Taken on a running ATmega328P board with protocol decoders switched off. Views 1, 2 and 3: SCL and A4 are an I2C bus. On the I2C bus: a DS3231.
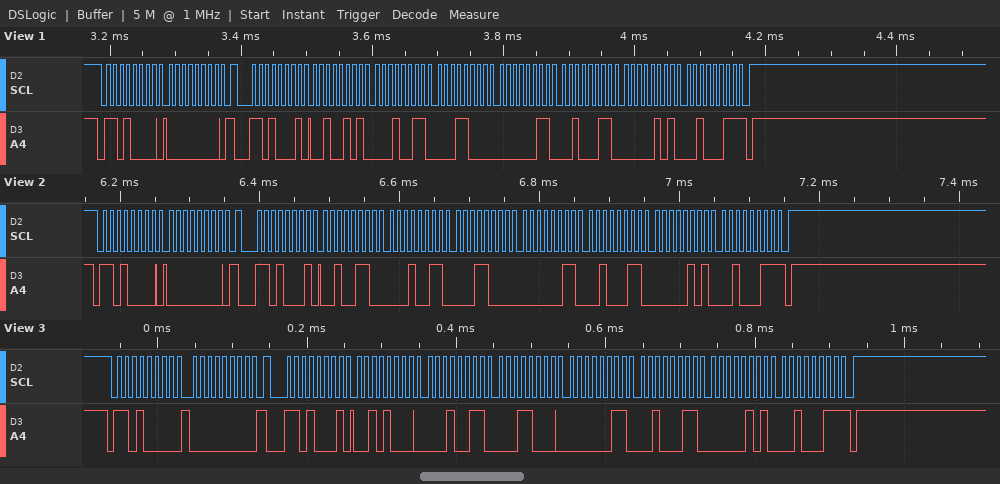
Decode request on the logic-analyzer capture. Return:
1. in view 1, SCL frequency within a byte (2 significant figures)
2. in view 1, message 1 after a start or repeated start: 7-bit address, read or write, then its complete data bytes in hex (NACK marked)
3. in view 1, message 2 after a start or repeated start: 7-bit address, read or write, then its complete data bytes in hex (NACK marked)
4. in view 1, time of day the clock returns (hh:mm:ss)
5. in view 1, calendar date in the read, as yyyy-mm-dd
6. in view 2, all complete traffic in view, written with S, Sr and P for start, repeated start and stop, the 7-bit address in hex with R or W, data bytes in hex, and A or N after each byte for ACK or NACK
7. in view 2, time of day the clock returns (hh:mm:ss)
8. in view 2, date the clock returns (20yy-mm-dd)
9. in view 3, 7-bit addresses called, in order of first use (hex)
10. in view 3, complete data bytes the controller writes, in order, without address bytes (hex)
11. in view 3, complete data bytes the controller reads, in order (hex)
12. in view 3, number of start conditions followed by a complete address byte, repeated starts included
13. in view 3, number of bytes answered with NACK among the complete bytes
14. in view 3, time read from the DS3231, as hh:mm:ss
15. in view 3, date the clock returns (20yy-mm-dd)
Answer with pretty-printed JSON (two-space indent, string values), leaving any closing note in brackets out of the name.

{
  "in view 1, SCL frequency within a byte": "100 kHz",
  "in view 1, message 1 after a start or repeated start: 7-bit address, read or write, then its complete data bytes in hex": "0x68 write: 00",
  "in view 1, message 2 after a start or repeated start: 7-bit address, read or write, then its complete data bytes in hex": "0x68 read: 25 13 18 03 23 05 23 NACK",
  "in view 1, time of day the clock returns": "18:13:25",
  "in view 1, calendar date in the read, as yyyy-mm-dd": "2023-05-23",
  "in view 2, all complete traffic in view, written with S, Sr and P for start, repeated start and stop, the 7-bit address in hex with R or W, data bytes in hex, and A or N after each byte for ACK or NACK": "S 68W A 00 A Sr 68R A 26 A 13 A 18 A 03 A 23 A 05 A 23 N P",
  "in view 2, time of day the clock returns": "18:13:26",
  "in view 2, date the clock returns": "2023-05-23",
  "in view 3, 7-bit addresses called, in order of first use": "0x68",
  "in view 3, complete data bytes the controller writes, in order, without address bytes": "00",
  "in view 3, complete data bytes the controller reads, in order": "28 13 18 03 23 05 23",
  "in view 3, number of start conditions followed by a complete address byte, repeated starts included": "2",
  "in view 3, number of bytes answered with NACK among the complete bytes": "1",
  "in view 3, time read from the DS3231, as hh:mm:ss": "18:13:28",
  "in view 3, date the clock returns": "2023-05-23"
}
